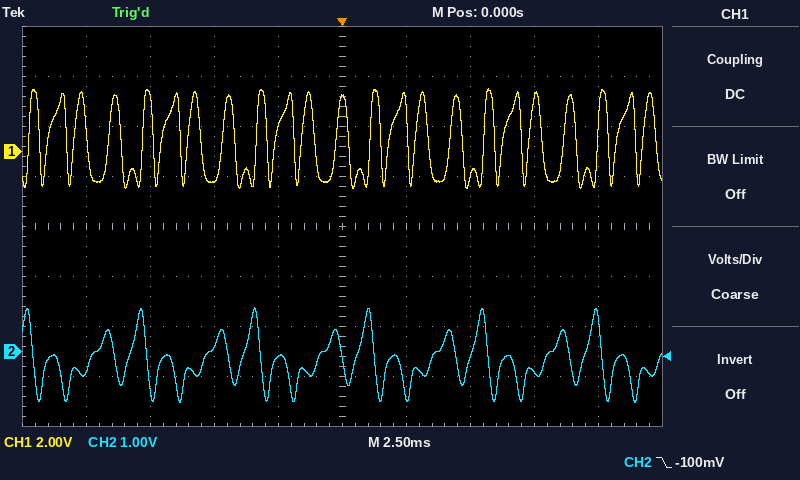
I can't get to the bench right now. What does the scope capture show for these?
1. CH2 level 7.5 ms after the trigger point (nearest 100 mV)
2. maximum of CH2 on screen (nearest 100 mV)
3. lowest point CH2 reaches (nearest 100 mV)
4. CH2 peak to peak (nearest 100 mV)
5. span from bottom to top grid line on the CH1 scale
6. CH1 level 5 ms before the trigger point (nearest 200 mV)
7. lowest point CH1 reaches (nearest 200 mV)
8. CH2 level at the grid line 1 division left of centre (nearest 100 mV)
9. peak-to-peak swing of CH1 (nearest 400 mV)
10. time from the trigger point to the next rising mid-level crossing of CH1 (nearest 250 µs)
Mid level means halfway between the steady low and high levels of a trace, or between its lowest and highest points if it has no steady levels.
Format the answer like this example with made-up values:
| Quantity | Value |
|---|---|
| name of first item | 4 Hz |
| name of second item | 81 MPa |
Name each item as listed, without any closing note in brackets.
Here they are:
| Quantity | Value |
|---|---|
| CH2 level 7.5 ms after the trigger point | -400 mV |
| maximum of CH2 on screen | 900 mV |
| lowest point CH2 reaches | -1.0 V |
| CH2 peak to peak | 1.9 V |
| span from bottom to top grid line on the CH1 scale | 16 V |
| CH1 level 5 ms before the trigger point | -1.2 V |
| lowest point CH1 reaches | -1.4 V |
| CH2 level at the grid line 1 division left of centre | -100 mV |
| peak-to-peak swing of CH1 | 4.0 V |
| time from the trigger point to the next rising mid-level crossing of CH1 | 1.00 ms |
